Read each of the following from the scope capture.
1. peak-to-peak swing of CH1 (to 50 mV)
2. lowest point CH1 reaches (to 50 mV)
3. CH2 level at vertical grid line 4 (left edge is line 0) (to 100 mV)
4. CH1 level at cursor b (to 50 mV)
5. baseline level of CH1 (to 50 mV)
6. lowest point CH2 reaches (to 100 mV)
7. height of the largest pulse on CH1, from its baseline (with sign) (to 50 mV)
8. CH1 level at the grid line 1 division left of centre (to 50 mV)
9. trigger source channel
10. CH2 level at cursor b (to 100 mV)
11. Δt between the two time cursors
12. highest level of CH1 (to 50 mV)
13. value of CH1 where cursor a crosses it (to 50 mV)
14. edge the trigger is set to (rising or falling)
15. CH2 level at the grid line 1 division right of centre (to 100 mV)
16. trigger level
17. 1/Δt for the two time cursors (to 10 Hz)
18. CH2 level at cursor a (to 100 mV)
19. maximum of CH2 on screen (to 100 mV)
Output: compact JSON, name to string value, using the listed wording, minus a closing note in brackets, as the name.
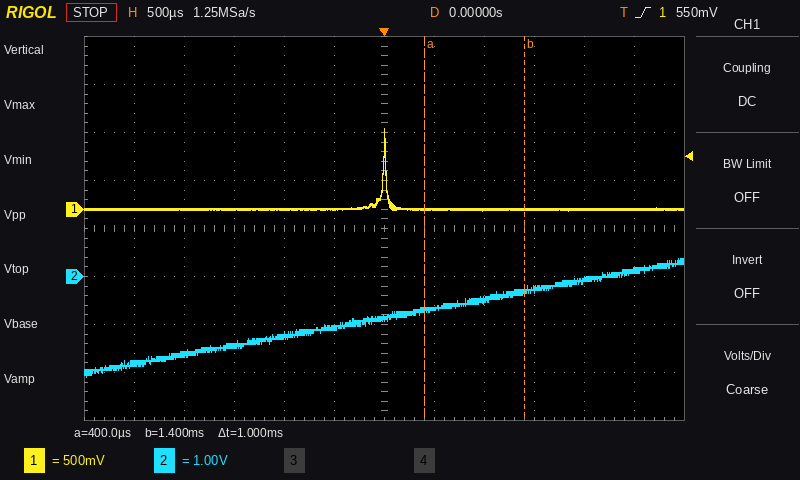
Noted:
{"peak-to-peak swing of CH1": "850 mV", "lowest point CH1 reaches": "0 mV", "CH2 level at vertical grid line 4 (left edge is line 0)": "-1.2 V", "CH1 level at cursor b": "0 mV", "baseline level of CH1": "0 mV", "lowest point CH2 reaches": "-2.1 V", "height of the largest pulse on CH1, from its baseline (with sign)": "+850 mV", "CH1 level at the grid line 1 division left of centre": "0 mV", "trigger source channel": "CH1", "CH2 level at cursor b": "-300 mV", "Δt between the two time cursors": "1 ms", "highest level of CH1": "850 mV", "value of CH1 where cursor a crosses it": "0 mV", "edge the trigger is set to": "rising", "CH2 level at the grid line 1 division right of centre": "-700 mV", "trigger level": "550 mV", "1/Δt for the two time cursors": "1.00 kHz", "CH2 level at cursor a": "-700 mV", "maximum of CH2 on screen": "400 mV"}
